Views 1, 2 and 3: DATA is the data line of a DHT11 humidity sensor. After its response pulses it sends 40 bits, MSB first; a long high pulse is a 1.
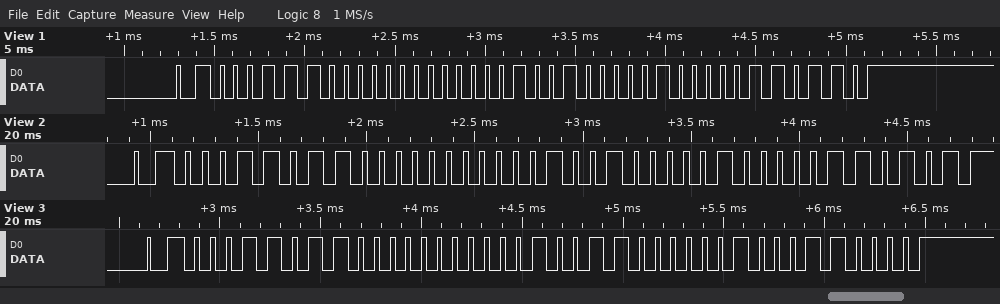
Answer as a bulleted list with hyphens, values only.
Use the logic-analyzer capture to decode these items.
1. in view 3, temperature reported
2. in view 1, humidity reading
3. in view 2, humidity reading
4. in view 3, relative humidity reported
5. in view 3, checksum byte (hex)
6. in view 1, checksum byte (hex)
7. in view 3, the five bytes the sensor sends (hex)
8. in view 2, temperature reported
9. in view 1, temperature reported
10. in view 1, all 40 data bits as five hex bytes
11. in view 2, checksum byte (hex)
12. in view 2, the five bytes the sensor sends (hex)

- 19.2 °C
- 28 %
- 27 %
- 27 %
- 0x30
- 0x36
- 1B 00 13 02 30
- 18.8 °C
- 18.8 °C
- 1C 00 12 08 36
- 0x35
- 1B 00 12 08 35
